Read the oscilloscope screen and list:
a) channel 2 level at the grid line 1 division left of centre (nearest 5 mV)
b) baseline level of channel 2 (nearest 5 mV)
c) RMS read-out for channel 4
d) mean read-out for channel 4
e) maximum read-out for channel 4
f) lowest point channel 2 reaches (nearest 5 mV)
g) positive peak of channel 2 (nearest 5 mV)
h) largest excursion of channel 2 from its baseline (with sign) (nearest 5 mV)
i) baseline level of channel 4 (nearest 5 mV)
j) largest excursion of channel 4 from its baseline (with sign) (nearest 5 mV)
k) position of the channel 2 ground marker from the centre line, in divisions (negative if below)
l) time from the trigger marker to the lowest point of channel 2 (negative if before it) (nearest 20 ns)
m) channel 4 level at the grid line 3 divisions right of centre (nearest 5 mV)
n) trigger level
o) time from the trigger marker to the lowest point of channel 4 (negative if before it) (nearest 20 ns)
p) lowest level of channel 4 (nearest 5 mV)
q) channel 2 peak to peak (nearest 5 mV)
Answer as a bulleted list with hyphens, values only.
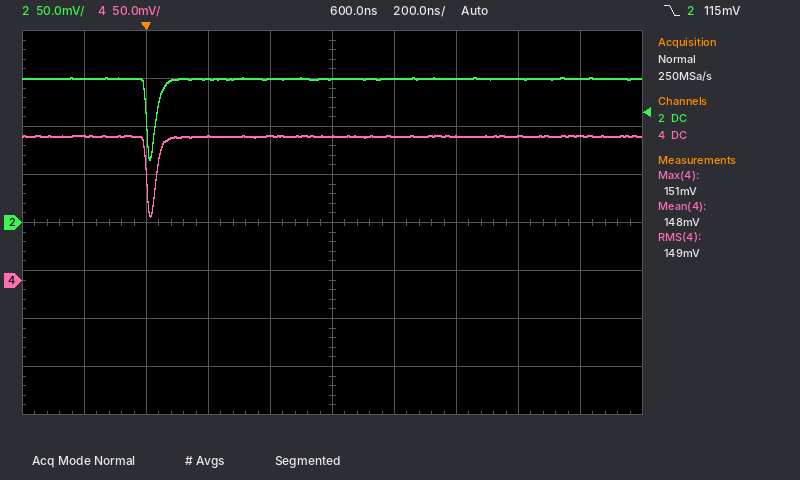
- 150 mV
- 150 mV
- 149 mV
- 148 mV
- 151 mV
- 65 mV
- 150 mV
- -85 mV
- 150 mV
- -85 mV
- 0.0 div
- +20 ns
- 150 mV
- 115 mV
- +20 ns
- 65 mV
- 85 mV
